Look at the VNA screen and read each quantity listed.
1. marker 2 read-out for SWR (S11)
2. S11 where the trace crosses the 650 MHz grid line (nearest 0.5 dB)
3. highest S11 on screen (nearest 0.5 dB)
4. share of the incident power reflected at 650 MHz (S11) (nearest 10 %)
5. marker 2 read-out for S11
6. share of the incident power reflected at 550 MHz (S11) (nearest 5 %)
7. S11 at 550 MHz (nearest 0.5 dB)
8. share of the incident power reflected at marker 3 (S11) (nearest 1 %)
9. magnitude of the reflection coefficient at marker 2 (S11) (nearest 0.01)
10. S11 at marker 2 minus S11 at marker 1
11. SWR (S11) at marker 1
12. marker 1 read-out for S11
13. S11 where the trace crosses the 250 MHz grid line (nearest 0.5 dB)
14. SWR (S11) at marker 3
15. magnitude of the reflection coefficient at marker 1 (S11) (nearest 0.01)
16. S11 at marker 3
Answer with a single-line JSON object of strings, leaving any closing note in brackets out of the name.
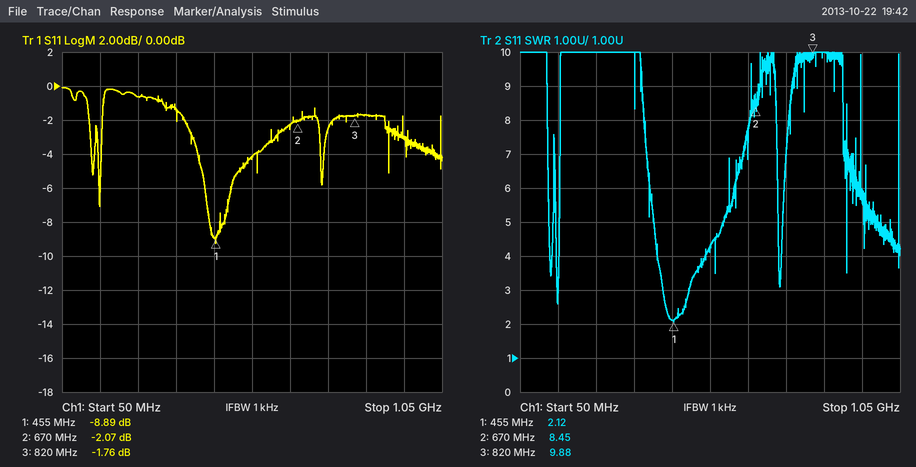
{"marker 2 read-out for SWR": "8.45", "S11 where the trace crosses the 650 MHz grid line": "-2.5 dB", "highest S11 on screen": "0.0 dB", "share of the incident power reflected at 650 MHz (S11)": "60 %", "marker 2 read-out for S11": "-2.07 dB", "share of the incident power reflected at 550 MHz (S11)": "40 %", "S11 at 550 MHz": "-4.0 dB", "share of the incident power reflected at marker 3 (S11)": "67 %", "magnitude of the reflection coefficient at marker 2 (S11)": "0.79", "S11 at marker 2 minus S11 at marker 1": "6.82 dB", "SWR (S11) at marker 1": "2.12", "marker 1 read-out for S11": "-8.89 dB", "S11 where the trace crosses the 250 MHz grid line": "-0.5 dB", "SWR (S11) at marker 3": "9.88", "magnitude of the reflection coefficient at marker 1 (S11)": "0.36", "S11 at marker 3": "-1.76 dB"}
